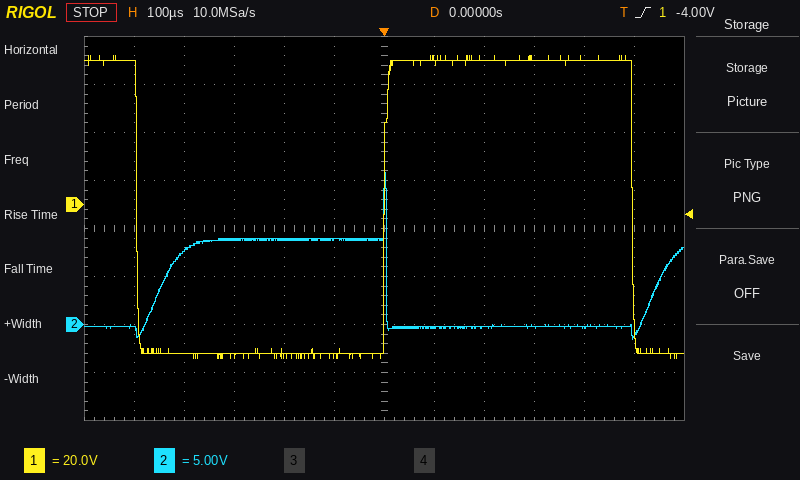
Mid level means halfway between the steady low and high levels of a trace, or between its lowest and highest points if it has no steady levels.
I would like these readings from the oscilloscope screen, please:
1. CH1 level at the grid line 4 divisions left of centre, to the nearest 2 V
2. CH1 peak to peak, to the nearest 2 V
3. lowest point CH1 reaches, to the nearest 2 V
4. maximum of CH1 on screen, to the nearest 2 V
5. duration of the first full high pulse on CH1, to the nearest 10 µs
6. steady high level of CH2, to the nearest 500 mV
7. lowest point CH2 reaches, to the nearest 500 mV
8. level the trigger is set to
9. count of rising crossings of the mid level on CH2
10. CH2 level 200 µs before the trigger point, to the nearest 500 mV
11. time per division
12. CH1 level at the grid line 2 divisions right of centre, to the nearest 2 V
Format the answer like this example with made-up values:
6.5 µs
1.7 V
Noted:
-62 V
126 V
-64 V
62 V
500 µs
9.0 V
-1.5 V
-4.00 V
2
9.0 V
100 µs
60 V
